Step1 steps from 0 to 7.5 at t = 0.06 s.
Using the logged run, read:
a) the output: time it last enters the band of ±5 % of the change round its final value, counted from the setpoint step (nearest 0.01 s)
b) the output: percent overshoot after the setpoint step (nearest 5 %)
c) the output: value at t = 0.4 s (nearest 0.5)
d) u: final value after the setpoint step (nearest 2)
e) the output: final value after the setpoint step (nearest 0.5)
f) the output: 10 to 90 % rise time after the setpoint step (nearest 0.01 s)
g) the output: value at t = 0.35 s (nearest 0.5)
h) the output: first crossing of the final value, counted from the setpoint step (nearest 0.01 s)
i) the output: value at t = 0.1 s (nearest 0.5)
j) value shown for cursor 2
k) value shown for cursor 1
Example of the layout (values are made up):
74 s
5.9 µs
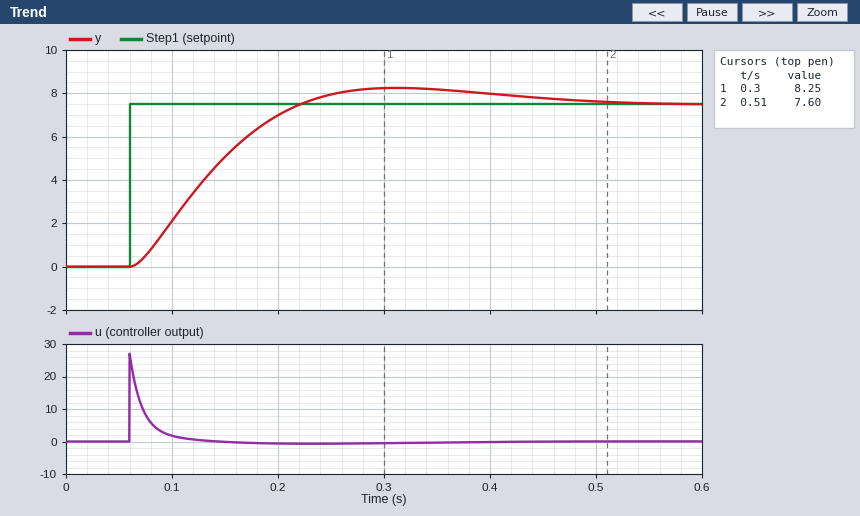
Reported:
0.36 s
10 %
8.0
0
7.5
0.11 s
8.0
0.16 s
2.0
7.60
8.25
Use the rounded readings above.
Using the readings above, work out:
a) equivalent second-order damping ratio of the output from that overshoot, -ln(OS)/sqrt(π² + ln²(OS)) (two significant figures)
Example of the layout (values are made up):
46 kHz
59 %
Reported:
0.59
